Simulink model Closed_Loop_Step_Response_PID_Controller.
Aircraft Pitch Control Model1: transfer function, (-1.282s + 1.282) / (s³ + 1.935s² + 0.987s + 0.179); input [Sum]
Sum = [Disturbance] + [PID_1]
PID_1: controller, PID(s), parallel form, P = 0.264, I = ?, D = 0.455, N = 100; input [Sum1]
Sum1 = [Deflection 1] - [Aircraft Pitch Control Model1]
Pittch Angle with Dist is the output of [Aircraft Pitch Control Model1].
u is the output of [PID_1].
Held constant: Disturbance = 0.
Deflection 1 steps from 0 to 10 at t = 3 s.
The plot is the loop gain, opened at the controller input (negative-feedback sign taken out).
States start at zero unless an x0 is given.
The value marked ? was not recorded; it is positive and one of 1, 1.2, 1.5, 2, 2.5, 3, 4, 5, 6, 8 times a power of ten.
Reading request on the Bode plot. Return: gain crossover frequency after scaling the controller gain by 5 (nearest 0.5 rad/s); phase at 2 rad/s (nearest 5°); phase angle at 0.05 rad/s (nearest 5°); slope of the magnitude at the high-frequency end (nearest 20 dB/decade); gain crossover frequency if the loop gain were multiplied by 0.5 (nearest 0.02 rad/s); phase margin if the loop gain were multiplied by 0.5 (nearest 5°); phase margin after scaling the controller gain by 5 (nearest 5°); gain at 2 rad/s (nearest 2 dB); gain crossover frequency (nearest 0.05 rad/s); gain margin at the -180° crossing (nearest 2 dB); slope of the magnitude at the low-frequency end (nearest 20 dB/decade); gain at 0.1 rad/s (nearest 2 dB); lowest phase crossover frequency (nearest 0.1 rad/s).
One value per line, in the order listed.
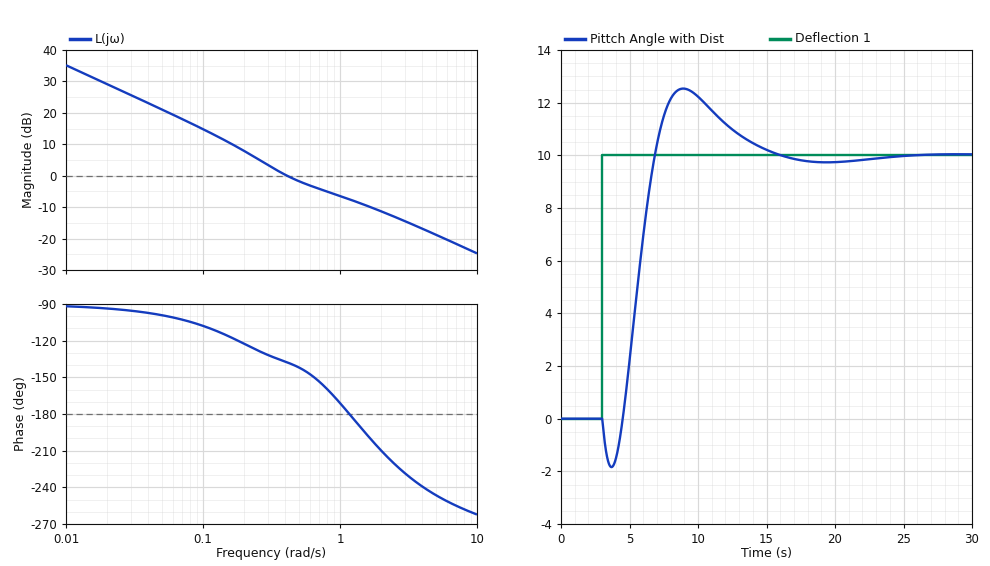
3.0 rad/s
-210°
-100°
-20 dB/decade
0.24 rad/s
55°
-45°
-12 dB
0.40 rad/s
8 dB
-20 dB/decade
14 dB
1.2 rad/s
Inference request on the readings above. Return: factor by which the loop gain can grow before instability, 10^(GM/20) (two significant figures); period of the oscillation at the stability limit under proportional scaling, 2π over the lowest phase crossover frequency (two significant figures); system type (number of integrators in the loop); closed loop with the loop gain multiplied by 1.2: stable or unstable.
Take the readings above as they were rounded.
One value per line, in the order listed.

2.5
5.2 s
1
stable
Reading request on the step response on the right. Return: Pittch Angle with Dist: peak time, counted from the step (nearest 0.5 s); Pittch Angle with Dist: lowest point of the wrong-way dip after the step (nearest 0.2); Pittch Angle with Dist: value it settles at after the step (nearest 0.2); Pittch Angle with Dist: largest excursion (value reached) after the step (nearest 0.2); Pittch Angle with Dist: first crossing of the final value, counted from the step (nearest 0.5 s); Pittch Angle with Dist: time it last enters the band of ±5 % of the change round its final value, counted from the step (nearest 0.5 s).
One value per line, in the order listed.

6.0 s
-1.8
10.0
12.6
4.0 s
11.0 s
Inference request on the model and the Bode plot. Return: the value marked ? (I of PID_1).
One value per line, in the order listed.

0.08
